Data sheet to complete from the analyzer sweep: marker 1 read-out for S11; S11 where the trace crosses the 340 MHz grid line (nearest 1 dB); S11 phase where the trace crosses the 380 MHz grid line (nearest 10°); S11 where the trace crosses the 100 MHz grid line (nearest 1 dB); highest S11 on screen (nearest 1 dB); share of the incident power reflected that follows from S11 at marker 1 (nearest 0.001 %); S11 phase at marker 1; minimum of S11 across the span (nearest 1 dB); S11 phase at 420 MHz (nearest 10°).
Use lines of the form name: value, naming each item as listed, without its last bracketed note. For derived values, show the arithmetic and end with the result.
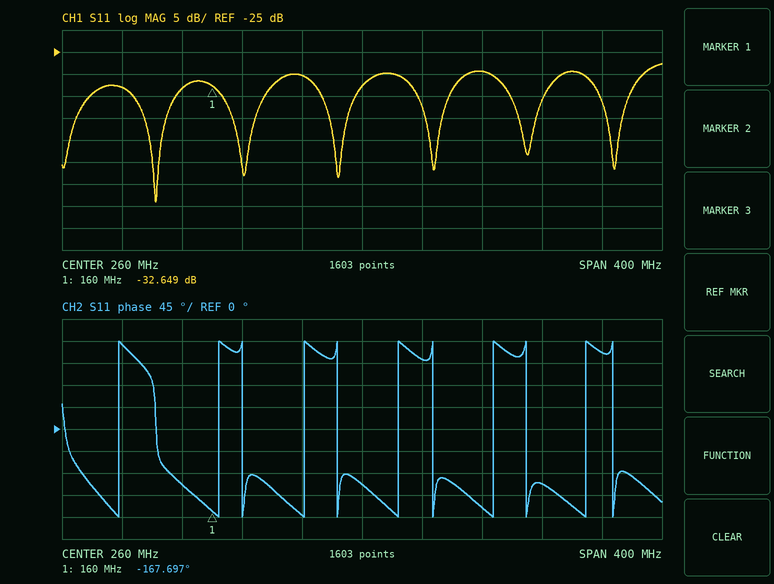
marker 1 read-out for S11: -32.649 dB
S11 where the trace crosses the 340 MHz grid line: -29 dB
S11 phase where the trace crosses the 380 MHz grid line: -110°
S11 where the trace crosses the 100 MHz grid line: -33 dB
highest S11 on screen: -28 dB
share of the incident power reflected that follows from S11 at marker 1: 10^(-32.649/10) ≈ 0.054 %
S11 phase at marker 1: -167.697°
minimum of S11 across the span: -59 dB
S11 phase at 420 MHz: 160°
